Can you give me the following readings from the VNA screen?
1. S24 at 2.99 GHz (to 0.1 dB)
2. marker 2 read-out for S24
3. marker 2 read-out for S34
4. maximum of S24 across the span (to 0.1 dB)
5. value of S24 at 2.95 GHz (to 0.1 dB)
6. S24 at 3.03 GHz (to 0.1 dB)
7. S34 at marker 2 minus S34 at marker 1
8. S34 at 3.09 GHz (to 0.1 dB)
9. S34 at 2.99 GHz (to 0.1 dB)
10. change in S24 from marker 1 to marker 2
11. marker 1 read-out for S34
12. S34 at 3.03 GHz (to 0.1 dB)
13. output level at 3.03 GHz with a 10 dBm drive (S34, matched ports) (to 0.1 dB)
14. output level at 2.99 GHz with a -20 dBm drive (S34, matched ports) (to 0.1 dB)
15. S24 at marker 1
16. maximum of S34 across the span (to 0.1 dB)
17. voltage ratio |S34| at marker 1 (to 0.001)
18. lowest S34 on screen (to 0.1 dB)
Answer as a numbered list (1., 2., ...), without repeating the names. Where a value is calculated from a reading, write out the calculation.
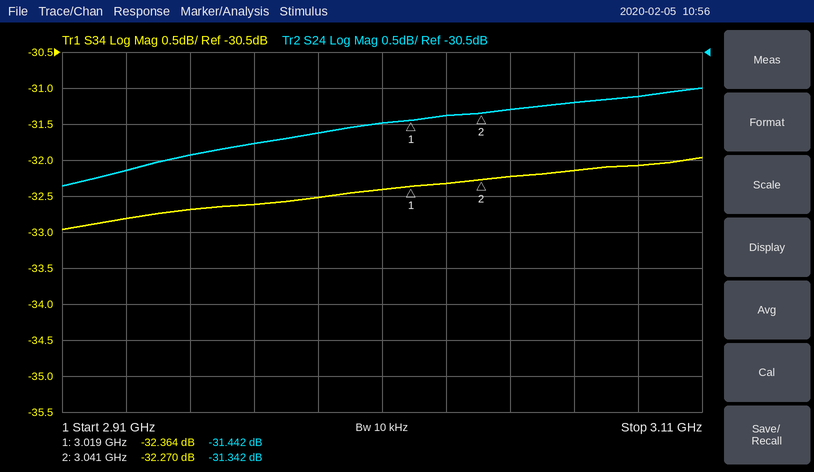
1. -31.6 dB
2. -31.342 dB
3. -32.270 dB
4. -31.0 dB
5. -31.9 dB
6. -31.4 dB
7. -32.27 − (-32.364) = 0.094 dB
8. -32.1 dB
9. -32.5 dB
10. -31.342 − (-31.442) = 0.100 dB
11. -32.364 dB
12. -32.3 dB
13. 10 dBm + (-32.3 dB) = -22.3 dBm
14. -20 dBm + (-32.5 dB) = -52.5 dBm
15. -31.442 dB
16. -32.0 dB
17. 10^(-32.364/20) ≈ 0.024
18. -33.0 dB
